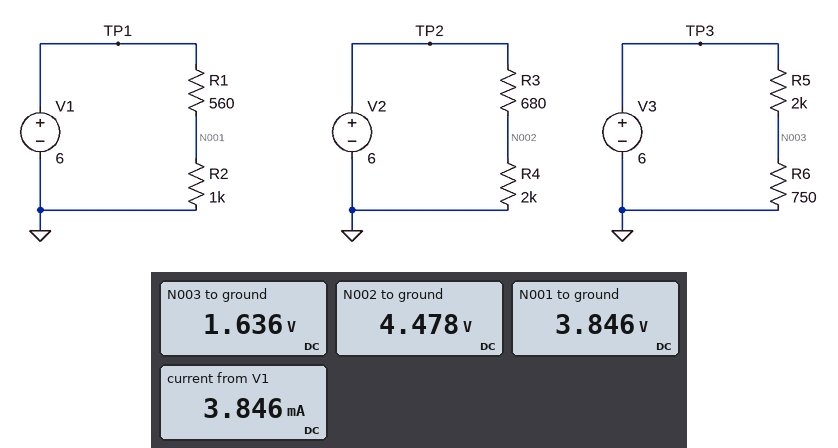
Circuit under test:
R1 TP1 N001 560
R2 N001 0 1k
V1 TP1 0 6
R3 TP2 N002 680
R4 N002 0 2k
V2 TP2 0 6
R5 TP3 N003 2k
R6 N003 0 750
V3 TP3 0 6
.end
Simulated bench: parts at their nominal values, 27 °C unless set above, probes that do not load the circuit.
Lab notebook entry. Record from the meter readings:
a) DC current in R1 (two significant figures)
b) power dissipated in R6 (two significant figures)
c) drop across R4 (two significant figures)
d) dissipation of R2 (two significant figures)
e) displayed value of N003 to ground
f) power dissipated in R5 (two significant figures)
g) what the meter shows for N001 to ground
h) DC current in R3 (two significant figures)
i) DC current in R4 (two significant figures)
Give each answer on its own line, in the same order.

3.8 mA
3.6 mW
4.5 V
15 mW
1.636 V
9.5 mW
3.846 V
2.2 mA
2.2 mA
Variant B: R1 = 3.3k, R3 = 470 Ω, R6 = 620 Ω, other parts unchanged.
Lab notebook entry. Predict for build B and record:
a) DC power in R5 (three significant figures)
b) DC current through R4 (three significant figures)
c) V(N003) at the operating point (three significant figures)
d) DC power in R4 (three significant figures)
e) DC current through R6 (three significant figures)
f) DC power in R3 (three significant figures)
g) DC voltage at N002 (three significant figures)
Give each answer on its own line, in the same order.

10.5 mW
2.43 mA
1.42 V
11.8 mW
2.29 mA
2.77 mW
4.86 V
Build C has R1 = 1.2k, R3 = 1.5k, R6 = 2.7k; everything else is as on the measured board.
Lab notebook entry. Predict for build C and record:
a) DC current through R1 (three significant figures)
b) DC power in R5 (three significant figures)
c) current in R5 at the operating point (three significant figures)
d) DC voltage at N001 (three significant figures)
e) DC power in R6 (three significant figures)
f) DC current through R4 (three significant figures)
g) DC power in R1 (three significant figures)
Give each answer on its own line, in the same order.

2.73 mA
3.26 mW
1.28 mA
2.73 V
4.40 mW
1.71 mA
8.93 mW
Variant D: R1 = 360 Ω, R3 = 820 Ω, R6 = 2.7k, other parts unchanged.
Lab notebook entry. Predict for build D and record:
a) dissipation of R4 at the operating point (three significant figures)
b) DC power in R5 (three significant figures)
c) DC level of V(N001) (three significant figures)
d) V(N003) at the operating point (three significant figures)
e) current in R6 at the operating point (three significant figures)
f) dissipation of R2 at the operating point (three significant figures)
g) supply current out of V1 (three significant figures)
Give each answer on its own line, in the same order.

9.05 mW
3.26 mW
4.41 V
3.45 V
1.28 mA
19.5 mW
4.41 mA
